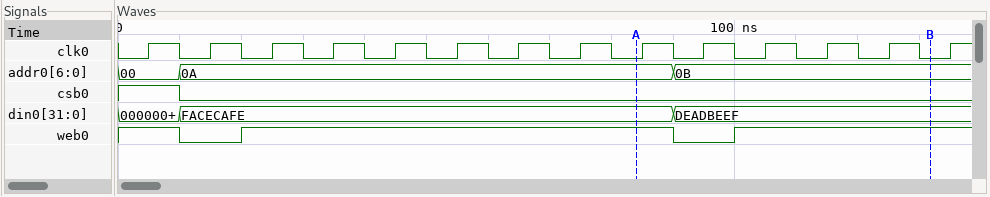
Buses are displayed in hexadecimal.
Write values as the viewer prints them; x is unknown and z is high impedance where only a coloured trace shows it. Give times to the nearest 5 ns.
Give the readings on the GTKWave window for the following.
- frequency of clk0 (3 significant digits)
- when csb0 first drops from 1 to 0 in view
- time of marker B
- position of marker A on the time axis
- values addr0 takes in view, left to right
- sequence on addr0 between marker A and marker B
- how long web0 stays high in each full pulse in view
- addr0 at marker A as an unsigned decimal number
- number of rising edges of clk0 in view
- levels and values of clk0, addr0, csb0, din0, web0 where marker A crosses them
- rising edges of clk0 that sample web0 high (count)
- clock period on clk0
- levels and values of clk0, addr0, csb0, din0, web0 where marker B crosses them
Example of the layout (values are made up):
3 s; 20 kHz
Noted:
100 MHz; 10 ns; 130 ns; 85 ns; 00, 0A, 0B; 0A, 0B; 70 ns; 10; 14; clk0=0, addr0=0A, csb0=0, din0=FACECAFE, web0=1; 12; 10 ns; clk0=0, addr0=0B, csb0=0, din0=DEADBEEF, web0=1
